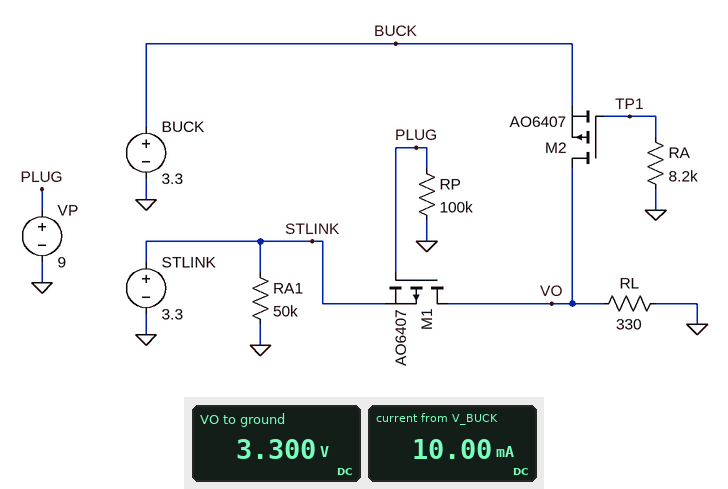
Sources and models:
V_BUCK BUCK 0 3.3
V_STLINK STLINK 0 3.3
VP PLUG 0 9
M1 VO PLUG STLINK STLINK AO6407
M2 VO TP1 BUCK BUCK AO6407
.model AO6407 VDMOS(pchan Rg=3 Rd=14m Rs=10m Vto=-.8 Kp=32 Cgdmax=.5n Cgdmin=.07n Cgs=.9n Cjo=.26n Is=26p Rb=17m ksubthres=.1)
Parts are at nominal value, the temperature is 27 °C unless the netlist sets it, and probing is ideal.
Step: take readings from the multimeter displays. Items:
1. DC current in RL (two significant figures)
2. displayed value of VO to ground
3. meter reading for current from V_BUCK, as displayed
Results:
10 mA
3.300 V
10.00 mA
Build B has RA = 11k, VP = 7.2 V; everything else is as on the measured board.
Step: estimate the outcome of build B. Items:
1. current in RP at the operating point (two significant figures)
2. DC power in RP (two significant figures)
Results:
72 µA
520 µW
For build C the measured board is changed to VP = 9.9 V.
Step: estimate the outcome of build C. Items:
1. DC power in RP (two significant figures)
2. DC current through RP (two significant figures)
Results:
980 µW
99 µA
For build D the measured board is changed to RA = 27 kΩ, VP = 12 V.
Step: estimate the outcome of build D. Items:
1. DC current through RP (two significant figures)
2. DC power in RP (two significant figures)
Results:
120 µA
1.4 mW
